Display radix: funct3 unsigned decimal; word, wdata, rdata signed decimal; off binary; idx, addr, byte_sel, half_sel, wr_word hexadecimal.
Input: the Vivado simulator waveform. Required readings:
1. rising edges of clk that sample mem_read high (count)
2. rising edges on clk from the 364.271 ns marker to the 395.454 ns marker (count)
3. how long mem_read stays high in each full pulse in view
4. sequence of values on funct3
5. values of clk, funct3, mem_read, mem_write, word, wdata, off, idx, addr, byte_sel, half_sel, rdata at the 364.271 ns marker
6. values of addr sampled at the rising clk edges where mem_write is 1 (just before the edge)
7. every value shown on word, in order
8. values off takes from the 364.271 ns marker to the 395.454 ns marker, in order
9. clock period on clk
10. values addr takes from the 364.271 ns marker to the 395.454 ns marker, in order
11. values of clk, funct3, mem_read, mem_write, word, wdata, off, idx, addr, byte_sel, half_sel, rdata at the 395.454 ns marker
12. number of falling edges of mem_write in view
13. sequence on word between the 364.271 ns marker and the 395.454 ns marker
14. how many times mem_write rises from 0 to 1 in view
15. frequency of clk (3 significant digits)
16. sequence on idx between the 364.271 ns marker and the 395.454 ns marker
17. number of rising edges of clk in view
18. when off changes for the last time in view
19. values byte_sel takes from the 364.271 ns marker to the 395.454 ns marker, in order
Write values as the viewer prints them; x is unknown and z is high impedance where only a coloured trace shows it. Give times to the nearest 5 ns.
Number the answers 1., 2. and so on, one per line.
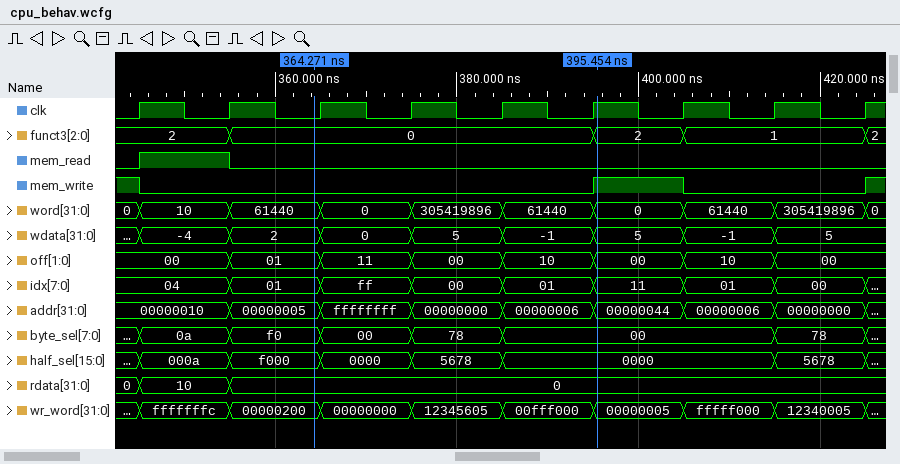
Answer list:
1. 1
2. 4
3. 10 ns
4. 2, 0, 2, 1, 2
5. clk=0, funct3=0, mem_read=0, mem_write=0, word=61440, wdata=2, off=01, idx=01, addr=00000005, byte_sel=f0, half_sel=f000, rdata=0
6. 00000010, 00000044
7. 0, 10, 61440, 0, 305419896, 61440, 0, 61440, 305419896, 0
8. 01, 11, 00, 10, 00
9. 10 ns
10. 00000005, ffffffff, 00000000, 00000006, 00000044
11. clk=1, funct3=2, mem_read=0, mem_write=1, word=0, wdata=5, off=00, idx=11, addr=00000044, byte_sel=00, half_sel=0000, rdata=0
12. 2
13. 61440, 0, 305419896, 61440, 0
14. 2
15. 100 MHz
16. 01, ff, 00, 01, 11
17. 9
18. 415 ns
19. f0, 00, 78, 00
